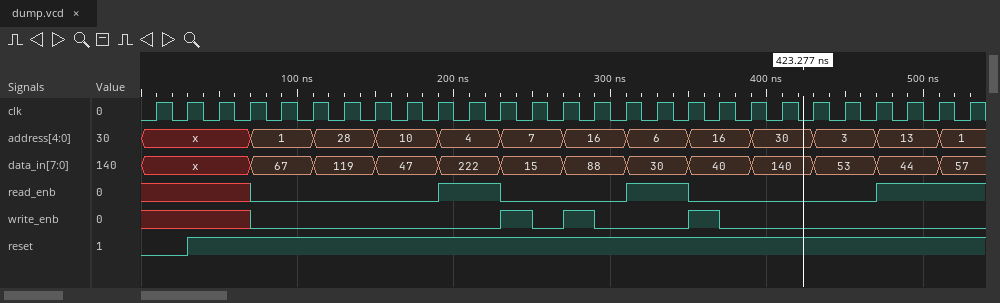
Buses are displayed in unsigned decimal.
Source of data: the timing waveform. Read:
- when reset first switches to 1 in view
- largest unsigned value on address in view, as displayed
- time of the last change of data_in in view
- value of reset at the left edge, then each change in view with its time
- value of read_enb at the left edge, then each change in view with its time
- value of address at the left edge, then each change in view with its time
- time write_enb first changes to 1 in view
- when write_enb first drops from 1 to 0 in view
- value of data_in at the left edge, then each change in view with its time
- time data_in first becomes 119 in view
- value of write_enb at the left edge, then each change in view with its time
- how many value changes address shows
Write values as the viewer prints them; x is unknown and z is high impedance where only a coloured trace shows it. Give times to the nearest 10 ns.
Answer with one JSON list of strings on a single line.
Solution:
["30 ns", "30", "510 ns", "0, 1 at 30 ns", "x, 0 at 70 ns, 1 at 190 ns, 0 at 230 ns, 1 at 310 ns, 0 at 350 ns, 1 at 470 ns", "x, 1 at 70 ns, 28 at 110 ns, 10 at 150 ns, 4 at 190 ns, 7 at 230 ns, 16 at 270 ns, 6 at 310 ns, 16 at 350 ns, 30 at 390 ns, 3 at 430 ns, 13 at 470 ns, 1 at 510 ns", "230 ns", "250 ns", "x, 67 at 70 ns, 119 at 110 ns, 47 at 150 ns, 222 at 190 ns, 15 at 230 ns, 88 at 270 ns, 30 at 310 ns, 40 at 350 ns, 140 at 390 ns, 53 at 430 ns, 44 at 470 ns, 57 at 510 ns", "110 ns", "x, 0 at 70 ns, 1 at 230 ns, 0 at 250 ns, 1 at 270 ns, 0 at 290 ns, 1 at 350 ns, 0 at 370 ns", "12"]
